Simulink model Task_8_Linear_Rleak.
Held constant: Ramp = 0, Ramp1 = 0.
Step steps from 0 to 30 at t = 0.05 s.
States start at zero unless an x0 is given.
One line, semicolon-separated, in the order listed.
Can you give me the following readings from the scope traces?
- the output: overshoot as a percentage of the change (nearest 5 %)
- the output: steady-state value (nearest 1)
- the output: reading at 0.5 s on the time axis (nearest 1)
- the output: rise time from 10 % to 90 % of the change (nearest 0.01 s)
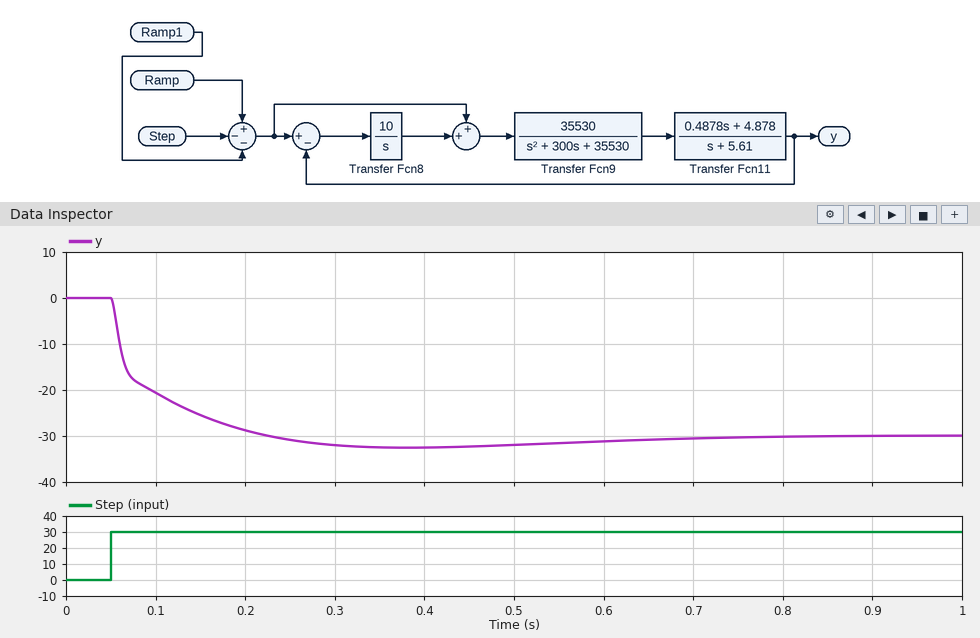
10 %; -30; -32; 0.12 s
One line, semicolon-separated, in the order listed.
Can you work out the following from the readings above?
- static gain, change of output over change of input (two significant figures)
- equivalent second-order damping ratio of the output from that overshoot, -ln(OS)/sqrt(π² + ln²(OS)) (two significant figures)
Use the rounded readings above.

-1.0; 0.59
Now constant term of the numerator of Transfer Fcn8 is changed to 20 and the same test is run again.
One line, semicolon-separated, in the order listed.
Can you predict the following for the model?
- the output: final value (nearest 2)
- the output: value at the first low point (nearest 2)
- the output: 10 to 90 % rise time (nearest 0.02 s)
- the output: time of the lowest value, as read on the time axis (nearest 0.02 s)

-30; -32; 0.08 s; 0.26 s
